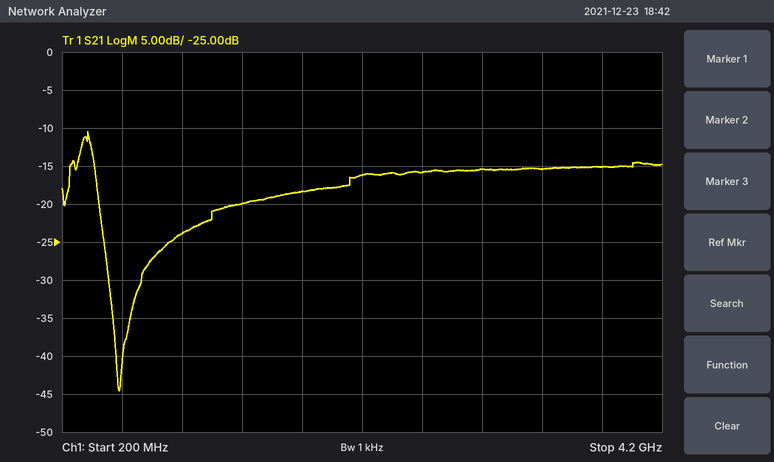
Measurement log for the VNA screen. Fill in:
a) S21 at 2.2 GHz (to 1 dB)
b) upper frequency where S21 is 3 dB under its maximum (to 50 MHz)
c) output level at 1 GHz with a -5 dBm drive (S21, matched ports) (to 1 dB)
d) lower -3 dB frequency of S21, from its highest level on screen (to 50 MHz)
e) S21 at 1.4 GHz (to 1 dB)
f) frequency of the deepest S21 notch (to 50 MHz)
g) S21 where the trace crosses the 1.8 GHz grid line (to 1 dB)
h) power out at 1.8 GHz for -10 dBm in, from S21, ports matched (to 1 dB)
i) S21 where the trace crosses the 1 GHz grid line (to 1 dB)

-16 dB
400 MHz
-29 dBm
300 MHz
-20 dB
600 MHz
-18 dB
-28 dBm
-24 dB
